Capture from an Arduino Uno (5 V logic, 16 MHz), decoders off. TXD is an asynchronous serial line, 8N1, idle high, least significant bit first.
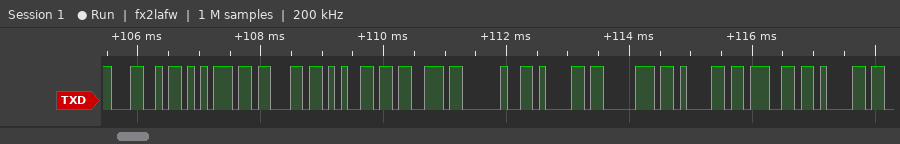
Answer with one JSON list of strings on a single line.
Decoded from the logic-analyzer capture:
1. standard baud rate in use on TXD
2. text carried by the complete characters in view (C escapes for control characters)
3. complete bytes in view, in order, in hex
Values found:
["9600 baud", "\"Luces apaga\"", "0x4C 0x75 0x63 0x65 0x73 0x20 0x61 0x70 0x61 0x67 0x61"]
